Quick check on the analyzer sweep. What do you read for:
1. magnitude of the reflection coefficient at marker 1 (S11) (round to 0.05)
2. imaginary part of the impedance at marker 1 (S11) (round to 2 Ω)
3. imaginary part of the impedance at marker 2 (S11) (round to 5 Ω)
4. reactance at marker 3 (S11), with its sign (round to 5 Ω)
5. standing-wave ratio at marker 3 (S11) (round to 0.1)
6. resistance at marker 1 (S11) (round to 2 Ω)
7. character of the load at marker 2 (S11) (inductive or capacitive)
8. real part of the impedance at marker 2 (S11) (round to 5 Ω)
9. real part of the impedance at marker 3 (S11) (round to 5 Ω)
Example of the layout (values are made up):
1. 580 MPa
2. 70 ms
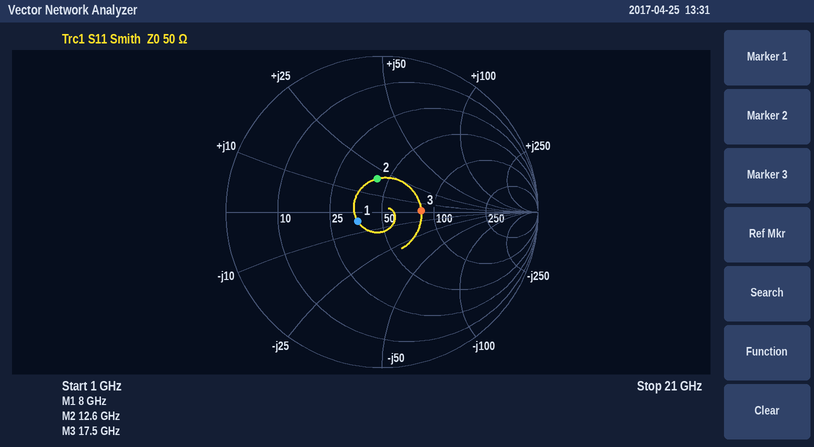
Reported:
1. 0.15
2. -4 Ω
3. +20 Ω
4. 0 Ω
5. 1.7
6. 36 Ω
7. inductive
8. 45 Ω
9. 85 Ω
